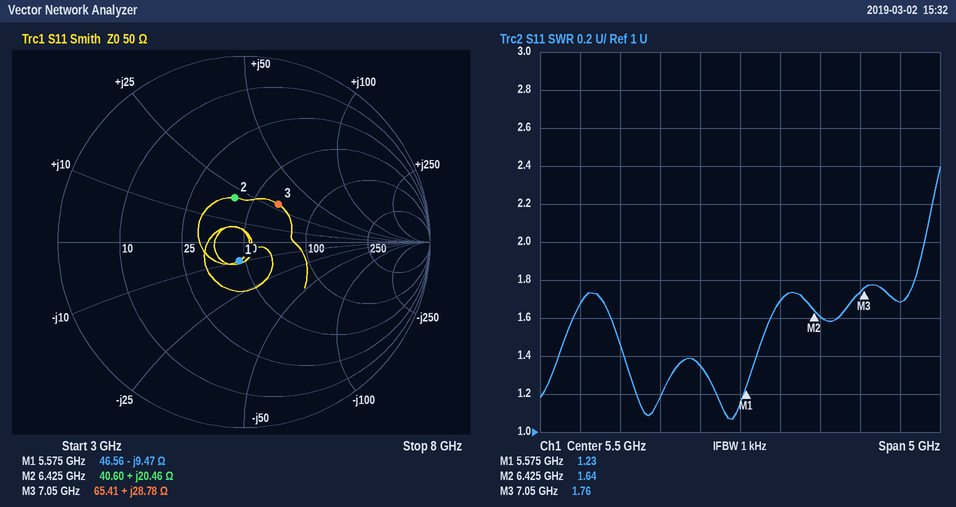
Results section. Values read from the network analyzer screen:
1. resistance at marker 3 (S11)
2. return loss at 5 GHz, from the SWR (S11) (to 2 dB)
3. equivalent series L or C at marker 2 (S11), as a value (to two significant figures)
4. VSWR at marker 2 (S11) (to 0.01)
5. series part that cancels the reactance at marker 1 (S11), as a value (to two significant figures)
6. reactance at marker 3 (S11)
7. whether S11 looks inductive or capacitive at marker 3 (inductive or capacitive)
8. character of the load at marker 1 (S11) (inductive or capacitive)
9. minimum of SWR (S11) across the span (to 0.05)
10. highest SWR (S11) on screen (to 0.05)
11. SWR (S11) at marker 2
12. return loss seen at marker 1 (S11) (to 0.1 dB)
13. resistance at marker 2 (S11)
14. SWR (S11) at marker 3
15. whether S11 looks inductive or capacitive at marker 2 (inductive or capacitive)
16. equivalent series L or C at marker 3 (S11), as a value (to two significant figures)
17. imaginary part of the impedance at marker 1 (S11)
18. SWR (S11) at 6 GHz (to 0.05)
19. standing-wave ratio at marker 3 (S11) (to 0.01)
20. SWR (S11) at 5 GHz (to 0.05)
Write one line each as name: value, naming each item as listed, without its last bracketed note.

resistance at marker 3: 65.41 Ω
return loss at 5 GHz, from the SWR (S11): 16 dB
equivalent series L or C at marker 2 (S11), as a value: 510 pH
VSWR at marker 2 (S11): 1.64
series part that cancels the reactance at marker 1 (S11), as a value: 270 pH
reactance at marker 3: +28.78 Ω
whether S11 looks inductive or capacitive at marker 3: inductive
character of the load at marker 1 (S11): capacitive
minimum of SWR (S11) across the span: 1.05
highest SWR (S11) on screen: 2.40
SWR (S11) at marker 2: 1.64
return loss seen at marker 1 (S11): 19.7 dB
resistance at marker 2: 40.60 Ω
SWR (S11) at marker 3: 1.76
whether S11 looks inductive or capacitive at marker 2: inductive
equivalent series L or C at marker 3 (S11), as a value: 650 pH
imaginary part of the impedance at marker 1: -9.47 Ω
SWR (S11) at 6 GHz: 1.70
standing-wave ratio at marker 3 (S11): 1.76
SWR (S11) at 5 GHz: 1.35
